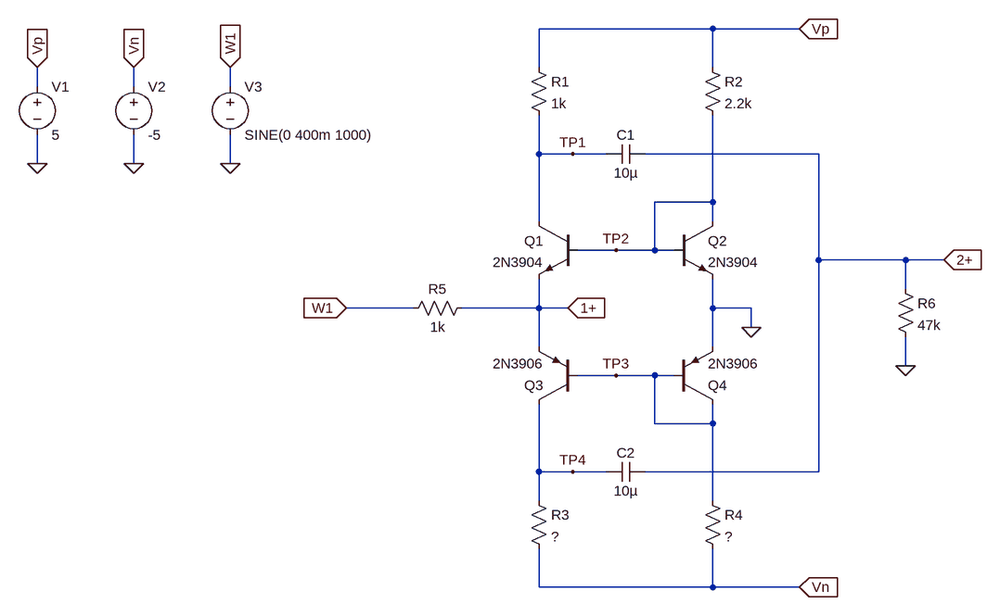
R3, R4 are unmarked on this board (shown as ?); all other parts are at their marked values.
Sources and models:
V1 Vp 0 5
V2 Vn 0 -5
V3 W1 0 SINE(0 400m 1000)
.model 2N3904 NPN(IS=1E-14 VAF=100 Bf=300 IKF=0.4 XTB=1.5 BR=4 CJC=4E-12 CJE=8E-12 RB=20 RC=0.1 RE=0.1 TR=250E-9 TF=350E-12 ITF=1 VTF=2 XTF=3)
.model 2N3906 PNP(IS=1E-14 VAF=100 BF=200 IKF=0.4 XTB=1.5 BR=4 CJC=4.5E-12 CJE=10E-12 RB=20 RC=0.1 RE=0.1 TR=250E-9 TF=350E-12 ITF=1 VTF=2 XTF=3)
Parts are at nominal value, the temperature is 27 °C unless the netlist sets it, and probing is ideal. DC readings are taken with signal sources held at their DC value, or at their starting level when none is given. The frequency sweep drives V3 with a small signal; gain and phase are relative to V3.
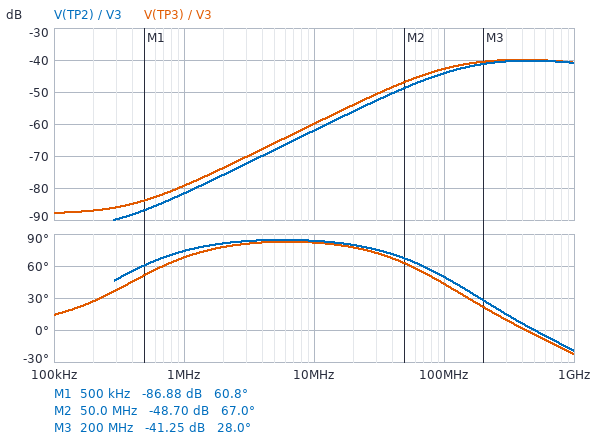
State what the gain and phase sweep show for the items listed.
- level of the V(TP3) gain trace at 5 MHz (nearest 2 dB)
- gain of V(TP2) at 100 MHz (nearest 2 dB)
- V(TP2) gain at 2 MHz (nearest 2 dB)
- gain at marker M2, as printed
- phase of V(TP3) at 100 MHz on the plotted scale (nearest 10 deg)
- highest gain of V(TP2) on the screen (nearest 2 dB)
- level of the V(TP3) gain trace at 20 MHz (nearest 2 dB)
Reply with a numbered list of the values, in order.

1. -66 dB
2. -44 dB
3. -76 dB
4. -48.70 dB
5. 40 deg
6. -40 dB
7. -54 dB
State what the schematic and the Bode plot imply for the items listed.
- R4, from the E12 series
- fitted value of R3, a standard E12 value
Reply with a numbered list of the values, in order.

1. 2.7 kΩ
2. 390 Ω
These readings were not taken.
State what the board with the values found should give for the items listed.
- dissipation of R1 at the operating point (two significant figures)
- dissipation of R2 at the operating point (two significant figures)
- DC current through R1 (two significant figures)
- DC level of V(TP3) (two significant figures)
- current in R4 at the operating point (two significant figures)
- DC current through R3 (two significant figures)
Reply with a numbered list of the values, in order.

1. 3.3 mW
2. 8.5 mW
3. 1.8 mA
4. -670 mV
5. 1.6 mA
6. 1.8 mA
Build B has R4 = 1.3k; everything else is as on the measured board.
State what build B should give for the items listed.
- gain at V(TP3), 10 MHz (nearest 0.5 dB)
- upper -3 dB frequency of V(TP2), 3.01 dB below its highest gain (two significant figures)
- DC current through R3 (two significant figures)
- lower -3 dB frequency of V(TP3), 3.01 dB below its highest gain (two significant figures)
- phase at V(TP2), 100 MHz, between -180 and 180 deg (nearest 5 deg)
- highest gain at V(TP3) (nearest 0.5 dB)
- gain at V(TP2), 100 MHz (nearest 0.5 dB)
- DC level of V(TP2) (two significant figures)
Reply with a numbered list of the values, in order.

1. -66.0 dB
2. 2.3 GHz
3. 2.6 mA
4. 170 MHz
5. 45 deg
6. -41.0 dB
7. -44.5 dB
8. 670 mV
